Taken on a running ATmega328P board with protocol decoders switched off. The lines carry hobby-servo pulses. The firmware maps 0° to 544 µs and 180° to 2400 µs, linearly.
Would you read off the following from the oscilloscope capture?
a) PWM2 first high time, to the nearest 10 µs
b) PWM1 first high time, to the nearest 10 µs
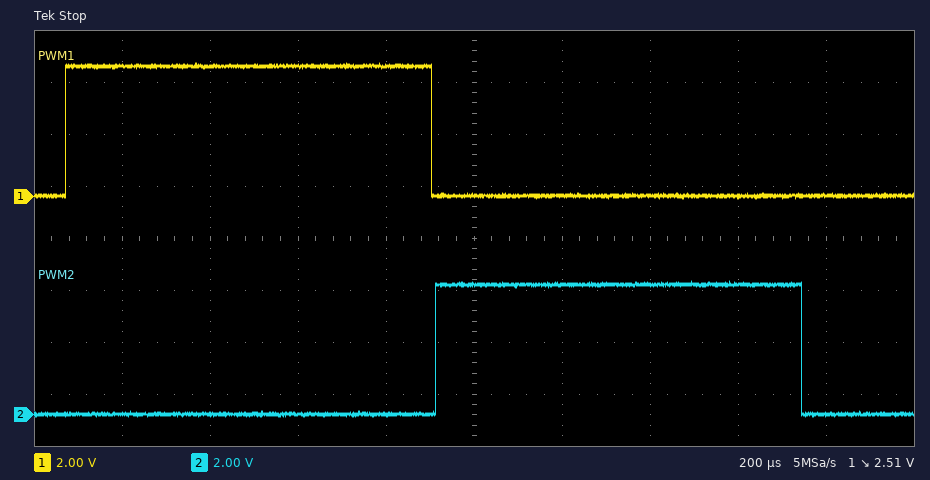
830 µs
830 µs
